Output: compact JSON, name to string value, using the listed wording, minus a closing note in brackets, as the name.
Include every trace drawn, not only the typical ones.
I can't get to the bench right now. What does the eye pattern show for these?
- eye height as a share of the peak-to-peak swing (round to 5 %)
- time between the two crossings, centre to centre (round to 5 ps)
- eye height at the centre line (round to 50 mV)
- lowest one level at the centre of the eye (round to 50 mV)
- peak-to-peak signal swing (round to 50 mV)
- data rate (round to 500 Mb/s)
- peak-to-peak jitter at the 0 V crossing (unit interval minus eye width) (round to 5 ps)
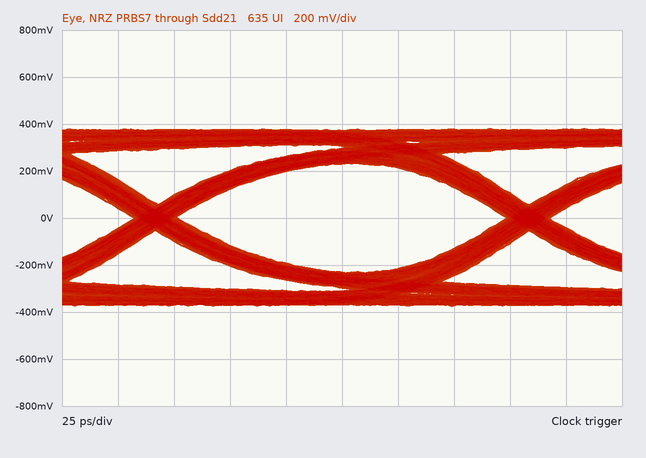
{"eye height as a share of the peak-to-peak swing": "60 %", "time between the two crossings, centre to centre": "165 ps", "eye height at the centre line": "450 mV", "lowest one level at the centre of the eye": "250 mV", "peak-to-peak signal swing": "750 mV", "data rate": "6.0 Gb/s", "peak-to-peak jitter at the 0 V crossing (unit interval minus eye width)": "20 ps"}
